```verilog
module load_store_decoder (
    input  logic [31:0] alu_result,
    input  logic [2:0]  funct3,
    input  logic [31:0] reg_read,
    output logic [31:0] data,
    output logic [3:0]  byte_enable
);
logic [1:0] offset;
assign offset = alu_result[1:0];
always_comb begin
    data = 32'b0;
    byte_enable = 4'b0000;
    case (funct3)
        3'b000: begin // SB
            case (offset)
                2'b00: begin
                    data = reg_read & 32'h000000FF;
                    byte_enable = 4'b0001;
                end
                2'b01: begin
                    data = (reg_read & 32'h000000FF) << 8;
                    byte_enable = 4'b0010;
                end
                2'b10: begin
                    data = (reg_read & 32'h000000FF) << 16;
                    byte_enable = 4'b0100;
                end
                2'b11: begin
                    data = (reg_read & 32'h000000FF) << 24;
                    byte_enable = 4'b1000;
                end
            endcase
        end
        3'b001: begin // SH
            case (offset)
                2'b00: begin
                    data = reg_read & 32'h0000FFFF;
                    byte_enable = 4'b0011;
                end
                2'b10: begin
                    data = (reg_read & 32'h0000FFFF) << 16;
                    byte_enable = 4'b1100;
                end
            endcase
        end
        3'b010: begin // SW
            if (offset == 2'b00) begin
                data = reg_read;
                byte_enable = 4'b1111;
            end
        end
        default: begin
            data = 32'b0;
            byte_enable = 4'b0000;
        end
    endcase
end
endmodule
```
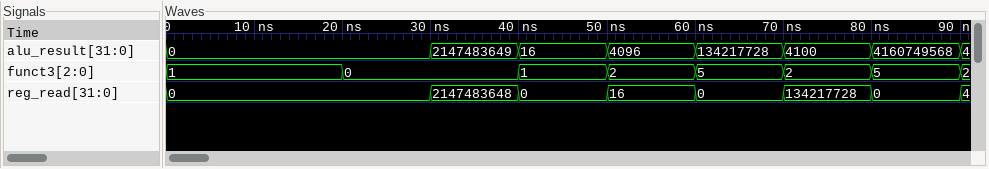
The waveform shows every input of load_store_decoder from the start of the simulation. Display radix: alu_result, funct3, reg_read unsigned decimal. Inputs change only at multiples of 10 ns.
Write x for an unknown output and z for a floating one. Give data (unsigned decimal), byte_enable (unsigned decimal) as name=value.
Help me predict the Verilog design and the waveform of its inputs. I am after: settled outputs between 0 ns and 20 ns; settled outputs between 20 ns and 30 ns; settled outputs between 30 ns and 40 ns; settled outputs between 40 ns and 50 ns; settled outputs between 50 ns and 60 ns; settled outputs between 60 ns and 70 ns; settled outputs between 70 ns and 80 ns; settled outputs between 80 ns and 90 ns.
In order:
data=0, byte_enable=3
data=0, byte_enable=1
data=0, byte_enable=2
data=0, byte_enable=3
data=16, byte_enable=15
data=0, byte_enable=0
data=134217728, byte_enable=15
data=0, byte_enable=0
